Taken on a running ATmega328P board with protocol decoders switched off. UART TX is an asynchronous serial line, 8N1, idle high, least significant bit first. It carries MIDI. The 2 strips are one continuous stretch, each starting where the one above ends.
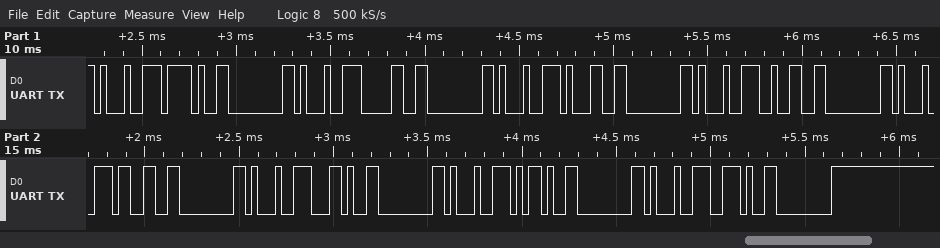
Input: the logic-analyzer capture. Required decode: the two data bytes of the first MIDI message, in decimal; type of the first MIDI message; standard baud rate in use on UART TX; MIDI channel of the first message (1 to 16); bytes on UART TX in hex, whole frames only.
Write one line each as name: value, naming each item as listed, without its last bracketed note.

the two data bytes of the first MIDI message, in decimal: 47, 0
type of the first MIDI message: Note On
standard baud rate in use on UART TX: 31250 baud
MIDI channel of the first message: 2
bytes on UART TX in hex, whole frames only: 0x91 0x2F 0x00 0x91 0x30 0x00 0x91 0x31 0x00 0x91 0x32 0x00 0x91 0x33 0x00 0x91 0x2C 0x00 0x91 0x2D 0x00 0x91 0x2E 0x00
